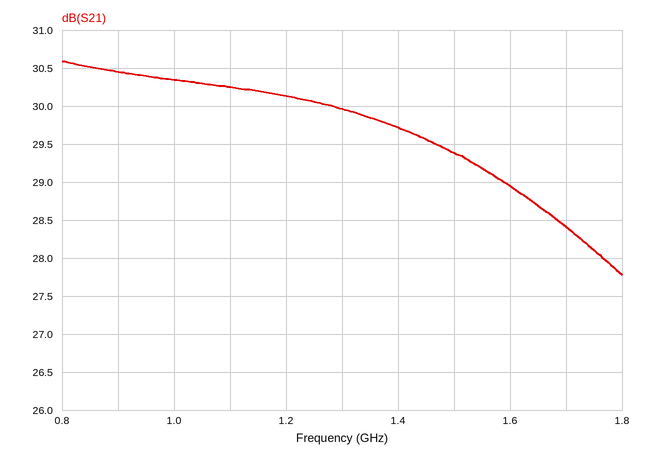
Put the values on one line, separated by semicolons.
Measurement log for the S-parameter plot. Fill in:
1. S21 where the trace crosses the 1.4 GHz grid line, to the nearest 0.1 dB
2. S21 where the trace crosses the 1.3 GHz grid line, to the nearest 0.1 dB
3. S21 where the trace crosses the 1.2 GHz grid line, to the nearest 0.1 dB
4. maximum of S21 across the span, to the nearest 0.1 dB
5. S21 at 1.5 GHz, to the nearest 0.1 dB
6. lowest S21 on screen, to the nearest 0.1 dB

29.7 dB; 30.0 dB; 30.1 dB; 30.6 dB; 29.4 dB; 27.8 dB
